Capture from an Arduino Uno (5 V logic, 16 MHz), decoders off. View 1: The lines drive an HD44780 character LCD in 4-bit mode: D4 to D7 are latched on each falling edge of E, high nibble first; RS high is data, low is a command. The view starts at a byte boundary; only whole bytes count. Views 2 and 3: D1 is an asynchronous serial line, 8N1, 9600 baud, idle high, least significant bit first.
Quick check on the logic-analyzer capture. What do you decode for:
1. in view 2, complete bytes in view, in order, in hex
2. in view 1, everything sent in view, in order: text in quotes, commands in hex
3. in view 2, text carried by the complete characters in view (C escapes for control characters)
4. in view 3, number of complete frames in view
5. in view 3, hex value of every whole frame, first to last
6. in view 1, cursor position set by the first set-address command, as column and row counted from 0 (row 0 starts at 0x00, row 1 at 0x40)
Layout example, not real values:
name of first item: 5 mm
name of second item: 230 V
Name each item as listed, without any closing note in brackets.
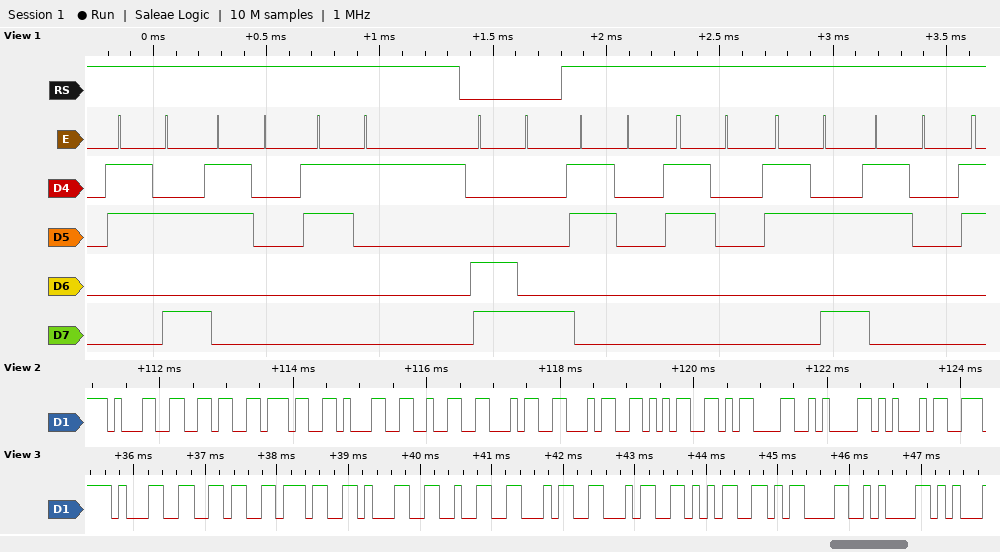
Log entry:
in view 2, complete bytes in view, in order, in hex: 31 36 37 31 32 34 34 35 0D 0A 45
in view 1, everything sent in view, in order: text in quotes, commands in hex: ":01" 0xC8 "00:0"
in view 2, text carried by the complete characters in view: "16712445\r\nE"
in view 3, number of complete frames in view: 10
in view 3, hex value of every whole frame, first to last: 0x31 0x36 0x37 0x31 0x32 0x34 0x34 0x35 0x0D 0x0A
in view 1, cursor position set by the first set-address command, as column and row counted from 0: column 8, row 1
